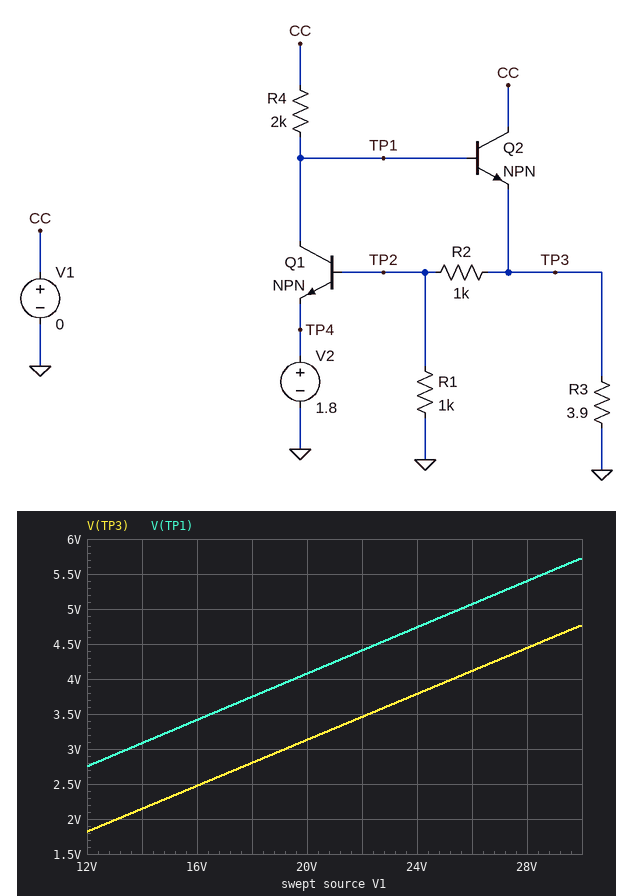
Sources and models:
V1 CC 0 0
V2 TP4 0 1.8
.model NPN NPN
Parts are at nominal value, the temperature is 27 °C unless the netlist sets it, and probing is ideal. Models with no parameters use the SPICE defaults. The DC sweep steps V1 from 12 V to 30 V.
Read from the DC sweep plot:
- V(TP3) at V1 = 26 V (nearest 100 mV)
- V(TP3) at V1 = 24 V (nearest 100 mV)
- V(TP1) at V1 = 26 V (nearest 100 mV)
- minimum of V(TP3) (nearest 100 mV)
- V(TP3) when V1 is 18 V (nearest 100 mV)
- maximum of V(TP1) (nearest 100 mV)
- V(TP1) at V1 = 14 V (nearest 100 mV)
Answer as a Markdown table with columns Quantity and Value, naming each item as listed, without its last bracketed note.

| Quantity | Value |
|---|---|
| V(TP3) at V1 = 26 V | 4.1 V |
| V(TP3) at V1 = 24 V | 3.8 V |
| V(TP1) at V1 = 26 V | 5.1 V |
| minimum of V(TP3) | 1.8 V |
| V(TP3) when V1 is 18 V | 2.8 V |
| maximum of V(TP1) | 5.7 V |
| V(TP1) at V1 = 14 V | 3.1 V |
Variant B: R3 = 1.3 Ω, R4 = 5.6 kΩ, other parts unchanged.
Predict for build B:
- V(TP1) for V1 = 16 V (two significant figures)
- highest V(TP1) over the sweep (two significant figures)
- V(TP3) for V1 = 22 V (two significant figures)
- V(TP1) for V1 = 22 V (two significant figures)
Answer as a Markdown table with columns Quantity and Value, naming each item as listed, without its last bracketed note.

| Quantity | Value |
|---|---|
| V(TP1) for V1 = 16 V | 1.3 V |
| highest V(TP1) over the sweep | 1.6 V |
| V(TP3) for V1 = 22 V | 480 mV |
| V(TP1) for V1 = 22 V | 1.4 V |
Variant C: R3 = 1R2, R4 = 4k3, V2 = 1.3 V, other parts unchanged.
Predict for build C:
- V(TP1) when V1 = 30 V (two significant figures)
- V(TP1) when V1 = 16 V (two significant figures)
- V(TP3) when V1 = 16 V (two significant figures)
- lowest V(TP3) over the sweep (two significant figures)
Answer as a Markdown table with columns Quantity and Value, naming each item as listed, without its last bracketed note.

| Quantity | Value |
|---|---|
| V(TP1) when V1 = 30 V | 1.7 V |
| V(TP1) when V1 = 16 V | 1.3 V |
| V(TP3) when V1 = 16 V | 410 mV |
| lowest V(TP3) over the sweep | 300 mV |
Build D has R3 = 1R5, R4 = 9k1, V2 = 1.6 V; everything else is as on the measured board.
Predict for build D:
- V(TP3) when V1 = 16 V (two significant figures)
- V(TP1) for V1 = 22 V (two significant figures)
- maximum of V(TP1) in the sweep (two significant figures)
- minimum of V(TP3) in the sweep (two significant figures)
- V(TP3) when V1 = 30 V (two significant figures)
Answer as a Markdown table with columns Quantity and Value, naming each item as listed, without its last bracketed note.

| Quantity | Value |
|---|---|
| V(TP3) when V1 = 16 V | 250 mV |
| V(TP1) for V1 = 22 V | 1.3 V |
| maximum of V(TP1) in the sweep | 1.4 V |
| minimum of V(TP3) in the sweep | 180 mV |
| V(TP3) when V1 = 30 V | 480 mV |
